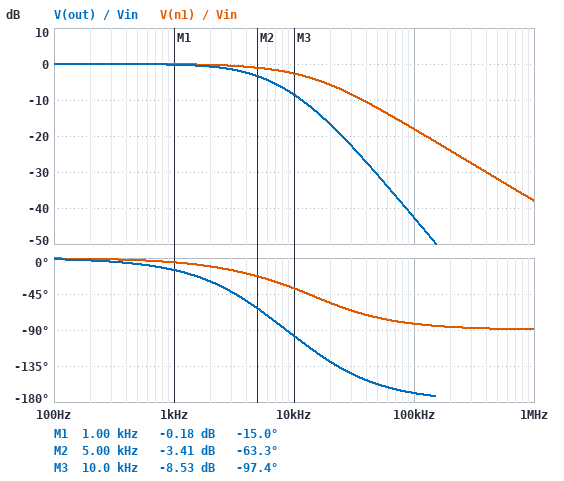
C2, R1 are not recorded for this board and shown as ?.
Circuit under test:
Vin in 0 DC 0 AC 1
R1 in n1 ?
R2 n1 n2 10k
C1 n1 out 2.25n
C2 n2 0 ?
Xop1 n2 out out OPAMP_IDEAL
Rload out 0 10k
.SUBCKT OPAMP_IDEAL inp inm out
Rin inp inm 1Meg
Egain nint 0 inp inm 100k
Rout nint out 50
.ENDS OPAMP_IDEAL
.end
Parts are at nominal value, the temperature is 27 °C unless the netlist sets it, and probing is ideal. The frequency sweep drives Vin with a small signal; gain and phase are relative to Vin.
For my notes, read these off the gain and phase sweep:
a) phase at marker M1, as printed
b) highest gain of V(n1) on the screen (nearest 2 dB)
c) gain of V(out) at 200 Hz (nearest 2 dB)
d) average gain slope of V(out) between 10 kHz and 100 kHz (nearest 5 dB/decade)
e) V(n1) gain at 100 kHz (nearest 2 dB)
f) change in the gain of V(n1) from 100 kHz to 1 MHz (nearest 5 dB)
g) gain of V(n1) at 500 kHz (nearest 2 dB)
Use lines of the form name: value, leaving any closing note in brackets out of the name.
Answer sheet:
phase at marker M1, as printed: -15.0 deg
highest gain of V(n1) on the screen: 0 dB
gain of V(out) at 200 Hz: 0 dB
average gain slope of V(out) between 10 kHz and 100 kHz: -35 dB/decade
V(n1) gain at 100 kHz: -18 dB
change in the gain of V(n1) from 100 kHz to 1 MHz: -20 dB
gain of V(n1) at 500 kHz: -32 dB
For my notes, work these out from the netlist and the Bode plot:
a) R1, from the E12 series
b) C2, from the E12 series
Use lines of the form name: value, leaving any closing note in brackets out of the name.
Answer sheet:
R1, from the E12 series: 5.6 kΩ
C2, from the E12 series: 2.7 nF
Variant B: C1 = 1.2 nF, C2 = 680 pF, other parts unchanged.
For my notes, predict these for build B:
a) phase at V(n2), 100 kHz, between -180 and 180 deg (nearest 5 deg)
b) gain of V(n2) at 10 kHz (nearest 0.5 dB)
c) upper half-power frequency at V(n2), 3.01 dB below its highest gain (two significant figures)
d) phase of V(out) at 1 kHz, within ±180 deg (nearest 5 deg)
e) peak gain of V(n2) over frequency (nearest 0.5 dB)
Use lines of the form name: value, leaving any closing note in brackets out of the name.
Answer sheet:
phase at V(n2), 100 kHz, between -180 and 180 deg: -160 deg
gain of V(n2) at 10 kHz: -0.5 dB
upper half-power frequency at V(n2), 3.01 dB below its highest gain: 21 kHz
phase of V(out) at 1 kHz, within ±180 deg: -5 deg
peak gain of V(n2) over frequency: 0 dB
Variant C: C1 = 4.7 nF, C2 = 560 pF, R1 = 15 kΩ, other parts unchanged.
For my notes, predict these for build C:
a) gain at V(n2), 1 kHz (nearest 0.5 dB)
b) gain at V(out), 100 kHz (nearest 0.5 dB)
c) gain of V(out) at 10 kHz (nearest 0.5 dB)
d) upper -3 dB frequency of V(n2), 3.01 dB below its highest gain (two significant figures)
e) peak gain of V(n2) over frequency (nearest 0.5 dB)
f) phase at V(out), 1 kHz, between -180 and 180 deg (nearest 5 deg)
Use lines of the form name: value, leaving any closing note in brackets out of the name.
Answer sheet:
gain at V(n2), 1 kHz: 0 dB
gain at V(out), 100 kHz: -44.0 dB
gain of V(out) at 10 kHz: -0.5 dB
upper -3 dB frequency of V(n2), 3.01 dB below its highest gain: 9.5 kHz
peak gain of V(n2) over frequency: 3.5 dB
phase at V(out), 1 kHz, between -180 and 180 deg: -5 deg
